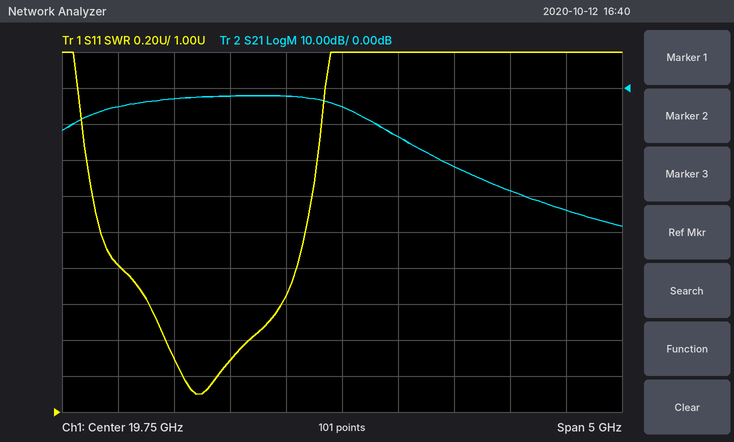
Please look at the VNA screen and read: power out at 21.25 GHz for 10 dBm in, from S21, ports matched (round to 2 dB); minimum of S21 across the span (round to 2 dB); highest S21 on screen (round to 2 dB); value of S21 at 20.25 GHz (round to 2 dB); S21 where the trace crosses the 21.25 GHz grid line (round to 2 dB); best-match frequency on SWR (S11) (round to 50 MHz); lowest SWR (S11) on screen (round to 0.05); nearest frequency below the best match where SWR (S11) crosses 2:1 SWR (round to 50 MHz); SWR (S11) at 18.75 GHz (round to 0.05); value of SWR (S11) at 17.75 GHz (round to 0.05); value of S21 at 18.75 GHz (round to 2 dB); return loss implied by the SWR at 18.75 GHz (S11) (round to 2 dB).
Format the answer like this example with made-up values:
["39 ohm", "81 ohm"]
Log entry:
["-18 dBm", "-38 dB", "-2 dB", "-14 dB", "-28 dB", "18.45 GHz", "1.10", "17.60 GHz", "1.30", "1.80", "-2 dB", "18 dB"]
